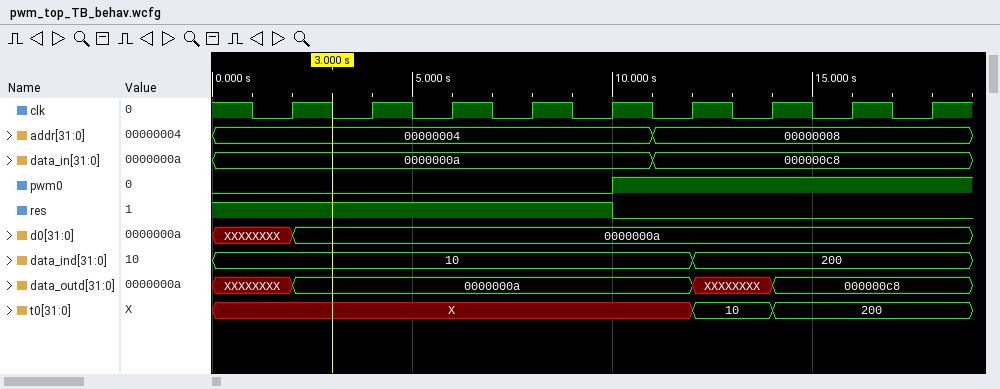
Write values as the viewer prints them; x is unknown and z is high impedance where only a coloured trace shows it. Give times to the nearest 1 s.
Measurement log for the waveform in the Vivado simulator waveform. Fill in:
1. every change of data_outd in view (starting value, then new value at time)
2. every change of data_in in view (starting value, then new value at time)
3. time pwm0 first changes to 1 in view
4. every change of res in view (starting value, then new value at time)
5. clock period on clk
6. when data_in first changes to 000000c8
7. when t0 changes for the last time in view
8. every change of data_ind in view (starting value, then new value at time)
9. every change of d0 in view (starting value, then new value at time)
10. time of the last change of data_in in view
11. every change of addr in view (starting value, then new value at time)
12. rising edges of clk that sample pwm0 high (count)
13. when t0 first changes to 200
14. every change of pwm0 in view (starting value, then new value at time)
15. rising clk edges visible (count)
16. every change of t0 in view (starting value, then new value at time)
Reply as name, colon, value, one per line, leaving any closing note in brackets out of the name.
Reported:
every change of data_outd in view: XXXXXXXX, 0000000a at 2 s, XXXXXXXX at 12 s, 000000c8 at 14 s
every change of data_in in view: 0000000a, 000000c8 at 11 s
time pwm0 first changes to 1 in view: 10 s
every change of res in view: 1, 0 at 10 s
clock period on clk: 2 s
when data_in first changes to 000000c8: 11 s
when t0 changes for the last time in view: 14 s
every change of data_ind in view: 10, 200 at 12 s
every change of d0 in view: XXXXXXXX, 0000000a at 2 s
time of the last change of data_in in view: 11 s
every change of addr in view: 00000004, 00000008 at 11 s
rising edges of clk that sample pwm0 high: 4
when t0 first changes to 200: 14 s
every change of pwm0 in view: 0, 1 at 10 s
rising clk edges visible: 9
every change of t0 in view: X, 10 at 12 s, 200 at 14 s
